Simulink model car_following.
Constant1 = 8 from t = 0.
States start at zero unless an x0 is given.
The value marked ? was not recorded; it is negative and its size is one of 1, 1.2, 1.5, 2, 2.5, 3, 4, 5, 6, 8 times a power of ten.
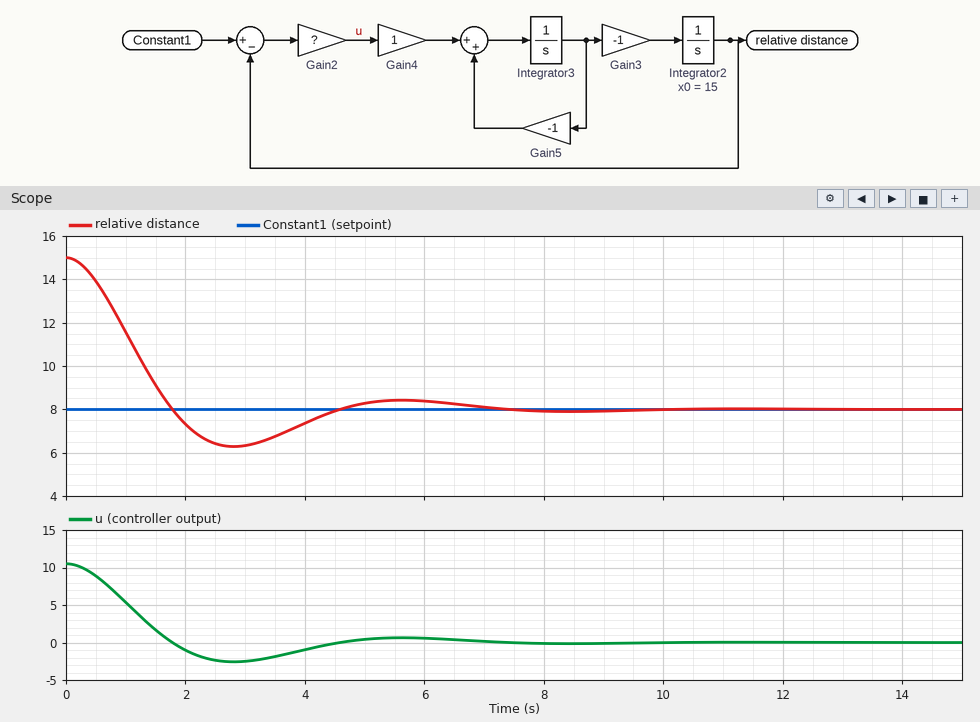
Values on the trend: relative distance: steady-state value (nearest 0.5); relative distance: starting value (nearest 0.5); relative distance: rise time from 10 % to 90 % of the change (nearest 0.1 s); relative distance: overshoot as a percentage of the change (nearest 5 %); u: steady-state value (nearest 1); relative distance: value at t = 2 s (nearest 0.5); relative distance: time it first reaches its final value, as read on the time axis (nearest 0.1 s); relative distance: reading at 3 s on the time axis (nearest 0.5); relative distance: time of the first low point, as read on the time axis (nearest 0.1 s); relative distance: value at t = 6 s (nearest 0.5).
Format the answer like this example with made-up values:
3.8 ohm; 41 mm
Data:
8.0; 15.0; 1.2 s; 25 %; 0; 7.5; 1.8 s; 6.5; 2.8 s; 8.5
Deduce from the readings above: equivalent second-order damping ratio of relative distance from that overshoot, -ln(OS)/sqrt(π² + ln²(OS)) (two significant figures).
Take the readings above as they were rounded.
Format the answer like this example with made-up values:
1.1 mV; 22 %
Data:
0.40
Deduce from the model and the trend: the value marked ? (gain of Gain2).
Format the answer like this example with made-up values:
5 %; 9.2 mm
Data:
-1.5
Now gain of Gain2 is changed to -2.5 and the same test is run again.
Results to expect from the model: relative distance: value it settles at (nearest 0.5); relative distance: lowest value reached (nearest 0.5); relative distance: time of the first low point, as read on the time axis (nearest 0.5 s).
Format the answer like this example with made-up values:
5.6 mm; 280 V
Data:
8.0; 5.5; 2.0 s
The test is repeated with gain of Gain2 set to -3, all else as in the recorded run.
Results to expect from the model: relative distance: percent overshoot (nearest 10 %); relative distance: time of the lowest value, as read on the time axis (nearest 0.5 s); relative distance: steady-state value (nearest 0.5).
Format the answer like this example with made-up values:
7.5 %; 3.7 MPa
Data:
40 %; 2.0 s; 8.0
